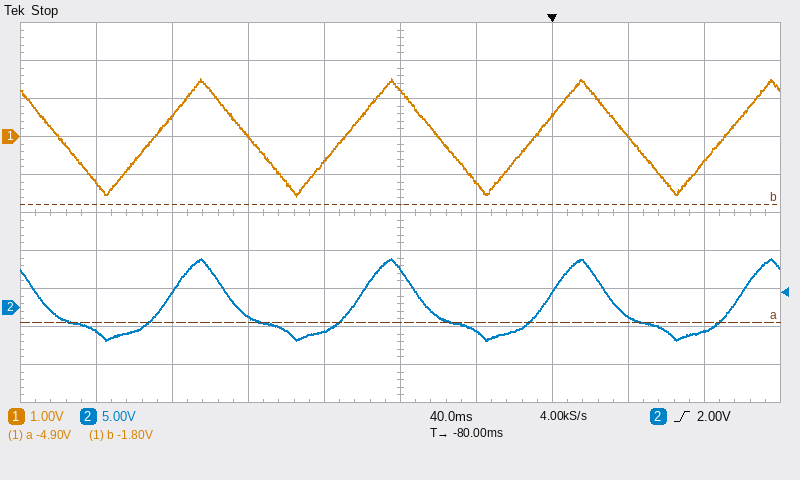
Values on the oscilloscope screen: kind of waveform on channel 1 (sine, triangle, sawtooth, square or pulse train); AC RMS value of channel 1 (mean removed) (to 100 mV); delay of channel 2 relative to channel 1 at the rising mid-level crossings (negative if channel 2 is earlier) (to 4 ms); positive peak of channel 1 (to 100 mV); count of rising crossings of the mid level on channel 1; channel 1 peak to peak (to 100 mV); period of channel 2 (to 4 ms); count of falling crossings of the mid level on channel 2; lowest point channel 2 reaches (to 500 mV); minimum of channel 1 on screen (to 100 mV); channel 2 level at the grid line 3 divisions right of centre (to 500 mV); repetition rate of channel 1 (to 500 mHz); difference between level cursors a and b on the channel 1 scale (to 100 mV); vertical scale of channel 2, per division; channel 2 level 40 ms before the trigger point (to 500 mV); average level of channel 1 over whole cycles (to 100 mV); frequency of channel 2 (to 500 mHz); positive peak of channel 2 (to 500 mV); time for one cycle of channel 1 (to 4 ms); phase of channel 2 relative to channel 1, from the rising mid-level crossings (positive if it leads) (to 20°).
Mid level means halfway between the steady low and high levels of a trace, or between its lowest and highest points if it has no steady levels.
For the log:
triangle
900 mV
+8 ms
1.5 V
4
3.1 V
100 ms
4
-4.5 V
-1.6 V
-1.0 V
10.0 Hz
3.1 V
5 V
-3.0 V
0.0 V
10.0 Hz
6.5 V
100 ms
-20°
